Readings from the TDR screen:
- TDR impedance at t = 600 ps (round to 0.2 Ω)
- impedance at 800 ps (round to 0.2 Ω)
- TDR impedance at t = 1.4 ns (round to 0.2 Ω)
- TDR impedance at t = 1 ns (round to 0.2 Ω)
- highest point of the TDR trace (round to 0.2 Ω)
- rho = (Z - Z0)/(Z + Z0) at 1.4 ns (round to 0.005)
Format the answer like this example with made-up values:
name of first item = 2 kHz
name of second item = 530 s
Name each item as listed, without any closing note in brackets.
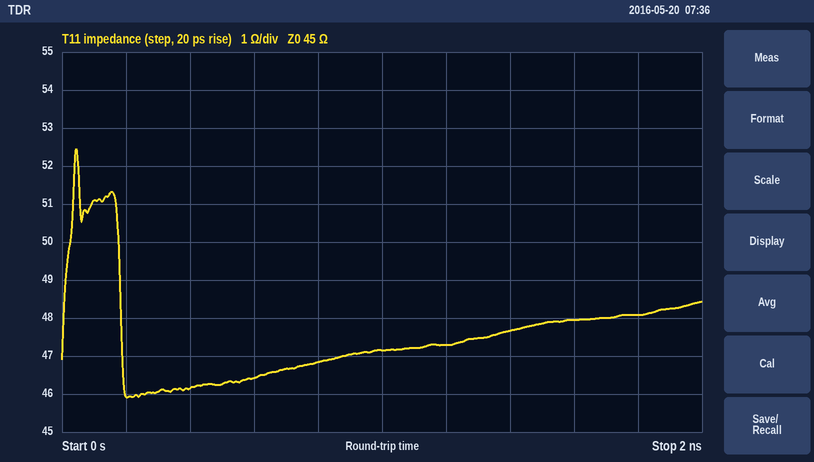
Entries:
TDR impedance at t = 600 ps = 46.4 Ω
impedance at 800 ps = 46.8 Ω
TDR impedance at t = 1.4 ns = 47.6 Ω
TDR impedance at t = 1 ns = 47.2 Ω
highest point of the TDR trace = 52.4 Ω
rho = (Z - Z0)/(Z + Z0) at 1.4 ns = +0.030
